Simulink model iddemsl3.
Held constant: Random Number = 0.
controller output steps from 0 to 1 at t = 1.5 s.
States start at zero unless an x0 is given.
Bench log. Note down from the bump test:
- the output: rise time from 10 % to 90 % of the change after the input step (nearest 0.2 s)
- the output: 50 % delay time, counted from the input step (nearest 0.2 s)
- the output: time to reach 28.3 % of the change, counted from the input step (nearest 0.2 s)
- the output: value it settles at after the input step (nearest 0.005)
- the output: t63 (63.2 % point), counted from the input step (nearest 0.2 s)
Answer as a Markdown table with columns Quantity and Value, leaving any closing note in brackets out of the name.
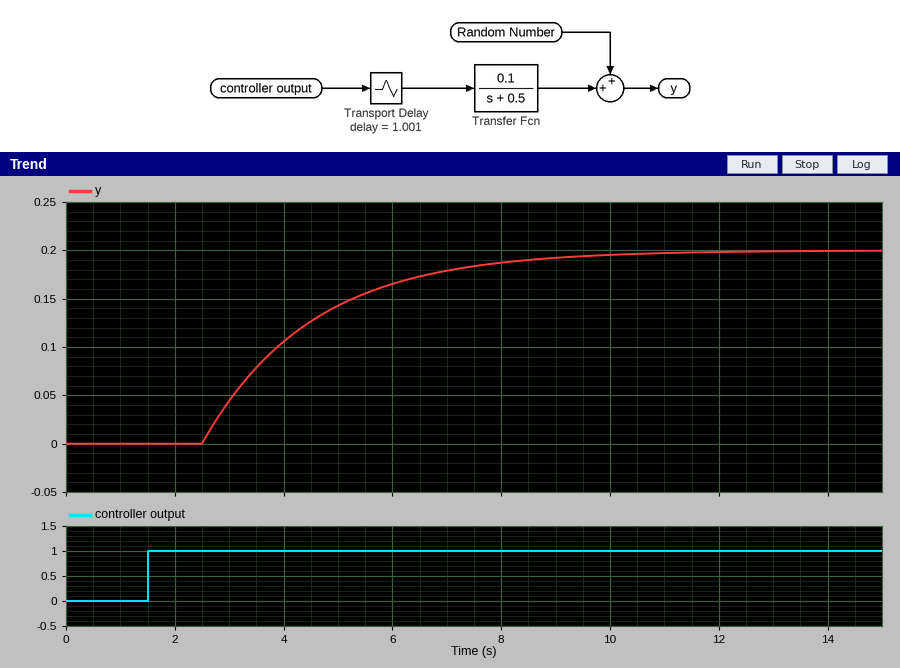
| Quantity | Value |
|---|---|
| the output: rise time from 10 % to 90 % of the change after the input step | 4.4 s |
| the output: 50 % delay time, counted from the input step | 2.4 s |
| the output: time to reach 28.3 % of the change, counted from the input step | 1.6 s |
| the output: value it settles at after the input step | 0.200 |
| the output: t63 (63.2 % point), counted from the input step | 3.0 s |
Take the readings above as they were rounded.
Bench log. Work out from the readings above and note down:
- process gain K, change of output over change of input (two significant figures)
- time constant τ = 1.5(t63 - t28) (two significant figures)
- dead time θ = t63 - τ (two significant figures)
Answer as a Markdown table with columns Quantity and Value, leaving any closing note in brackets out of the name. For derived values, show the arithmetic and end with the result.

| Quantity | Value |
|---|---|
| process gain K, change of output over change of input | (0.2 - 0) / 1 = 0.20 |
| time constant τ = 1.5(t63 - t28) | 1.5 × (3 - 1.6) = 2.1 s |
| dead time θ = t63 - τ | 3 - 2.1 = 0.90 s |
